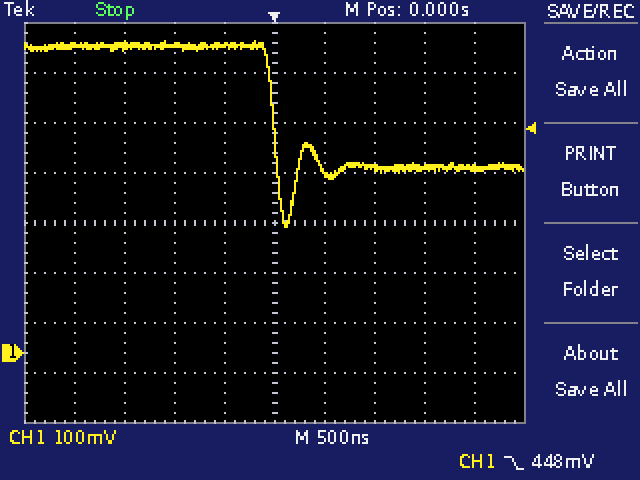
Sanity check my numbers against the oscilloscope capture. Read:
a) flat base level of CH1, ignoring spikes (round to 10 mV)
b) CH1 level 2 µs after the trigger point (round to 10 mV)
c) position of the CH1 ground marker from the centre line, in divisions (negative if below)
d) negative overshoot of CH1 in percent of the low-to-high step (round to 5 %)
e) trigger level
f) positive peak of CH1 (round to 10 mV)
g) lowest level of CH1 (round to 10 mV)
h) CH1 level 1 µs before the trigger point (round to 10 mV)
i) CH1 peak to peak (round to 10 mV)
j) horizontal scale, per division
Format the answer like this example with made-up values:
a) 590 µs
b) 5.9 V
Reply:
a) 370 mV
b) 370 mV
c) -2.6 div
d) 50 %
e) 448 mV
f) 620 mV
g) 250 mV
h) 620 mV
i) 370 mV
j) 500 ns
